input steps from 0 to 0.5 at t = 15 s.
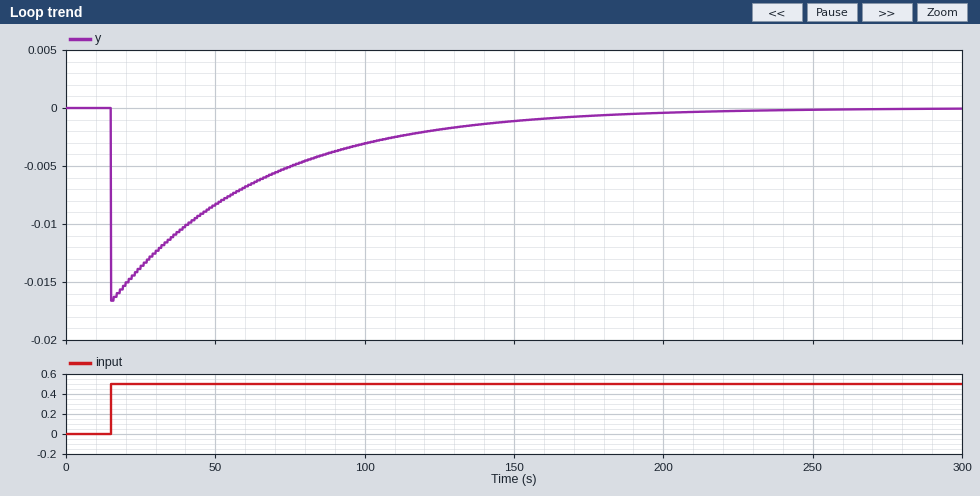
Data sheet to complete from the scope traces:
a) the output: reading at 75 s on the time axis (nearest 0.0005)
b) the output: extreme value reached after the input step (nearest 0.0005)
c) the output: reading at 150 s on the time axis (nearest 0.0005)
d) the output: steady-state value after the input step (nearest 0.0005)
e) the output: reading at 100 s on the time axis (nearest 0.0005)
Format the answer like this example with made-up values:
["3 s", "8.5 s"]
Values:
["-0.0050", "-0.0165", "-0.0010", "0.0000", "-0.0030"]
